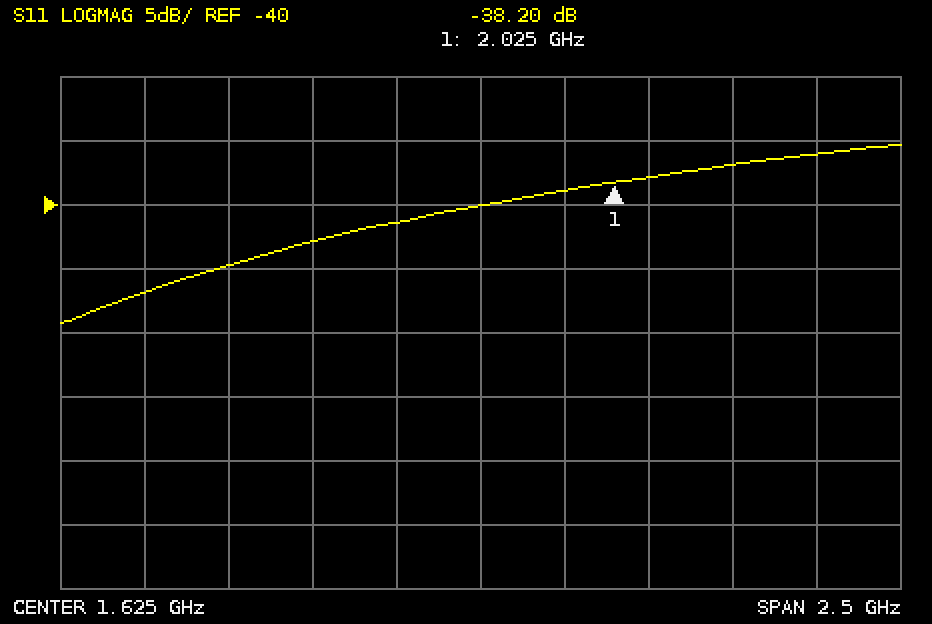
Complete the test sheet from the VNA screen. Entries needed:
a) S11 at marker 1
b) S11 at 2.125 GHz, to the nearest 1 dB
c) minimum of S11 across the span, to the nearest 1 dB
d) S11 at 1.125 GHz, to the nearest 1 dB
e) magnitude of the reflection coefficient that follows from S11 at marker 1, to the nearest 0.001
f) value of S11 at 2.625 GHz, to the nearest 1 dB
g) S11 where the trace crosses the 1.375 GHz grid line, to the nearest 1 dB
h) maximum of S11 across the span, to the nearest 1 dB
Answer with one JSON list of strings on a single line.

["-38.20 dB", "-38 dB", "-49 dB", "-43 dB", "0.012", "-36 dB", "-41 dB", "-35 dB"]
